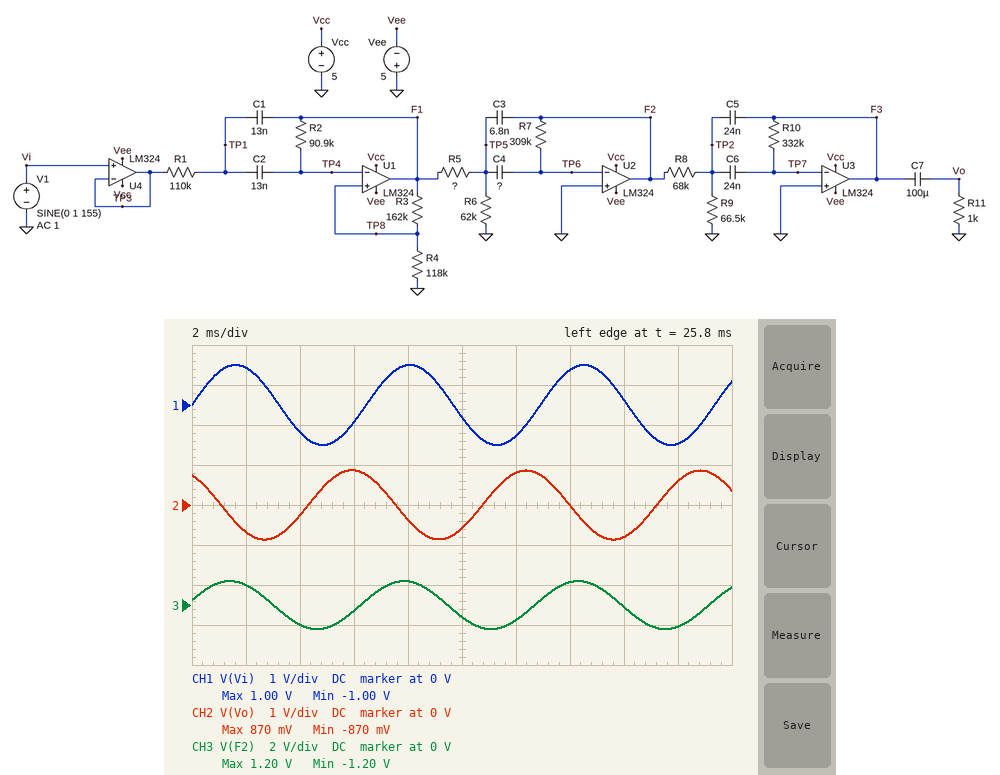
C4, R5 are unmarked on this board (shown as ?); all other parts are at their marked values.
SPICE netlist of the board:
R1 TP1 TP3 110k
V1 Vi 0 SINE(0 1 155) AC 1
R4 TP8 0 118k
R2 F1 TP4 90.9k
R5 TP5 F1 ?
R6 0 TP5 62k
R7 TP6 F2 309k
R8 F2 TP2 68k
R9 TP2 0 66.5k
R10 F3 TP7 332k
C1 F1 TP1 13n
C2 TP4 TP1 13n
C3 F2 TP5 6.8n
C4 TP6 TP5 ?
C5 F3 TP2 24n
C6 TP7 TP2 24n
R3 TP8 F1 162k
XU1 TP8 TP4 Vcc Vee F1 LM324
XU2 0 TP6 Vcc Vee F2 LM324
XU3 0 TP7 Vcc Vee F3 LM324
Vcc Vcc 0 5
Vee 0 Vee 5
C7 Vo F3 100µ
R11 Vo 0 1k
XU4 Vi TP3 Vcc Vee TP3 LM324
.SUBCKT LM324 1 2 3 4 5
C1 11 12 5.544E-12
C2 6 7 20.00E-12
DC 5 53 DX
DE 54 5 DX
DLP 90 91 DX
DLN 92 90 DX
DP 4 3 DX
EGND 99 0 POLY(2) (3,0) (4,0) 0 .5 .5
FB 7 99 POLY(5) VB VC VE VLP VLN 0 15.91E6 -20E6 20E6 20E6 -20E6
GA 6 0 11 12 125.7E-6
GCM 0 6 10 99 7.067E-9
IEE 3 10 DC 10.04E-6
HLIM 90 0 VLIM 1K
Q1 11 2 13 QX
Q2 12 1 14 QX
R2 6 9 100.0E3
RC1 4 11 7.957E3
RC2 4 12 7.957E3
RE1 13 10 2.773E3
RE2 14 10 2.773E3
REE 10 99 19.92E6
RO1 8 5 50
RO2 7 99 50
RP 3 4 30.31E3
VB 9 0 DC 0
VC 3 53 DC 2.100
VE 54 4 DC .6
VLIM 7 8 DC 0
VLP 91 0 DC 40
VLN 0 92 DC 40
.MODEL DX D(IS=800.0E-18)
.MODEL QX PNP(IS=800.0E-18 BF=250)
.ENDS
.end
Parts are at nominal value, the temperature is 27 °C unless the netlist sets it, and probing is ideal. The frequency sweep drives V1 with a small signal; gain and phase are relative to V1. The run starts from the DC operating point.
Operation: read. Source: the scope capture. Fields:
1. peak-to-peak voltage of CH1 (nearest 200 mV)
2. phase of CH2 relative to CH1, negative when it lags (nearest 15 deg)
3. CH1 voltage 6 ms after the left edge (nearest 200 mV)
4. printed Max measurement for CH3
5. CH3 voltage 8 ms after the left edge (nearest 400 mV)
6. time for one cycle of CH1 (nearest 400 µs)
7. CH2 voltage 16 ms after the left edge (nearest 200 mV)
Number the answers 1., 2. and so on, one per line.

1. 2.0 V
2. 120 deg
3. -400 mV
4. 1.20 V
5. 1.2 V
6. 6.4 ms
7. -800 mV
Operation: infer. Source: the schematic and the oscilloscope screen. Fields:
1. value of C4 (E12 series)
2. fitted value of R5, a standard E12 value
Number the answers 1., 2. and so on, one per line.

1. 8.2 nF
2. 120 kΩ
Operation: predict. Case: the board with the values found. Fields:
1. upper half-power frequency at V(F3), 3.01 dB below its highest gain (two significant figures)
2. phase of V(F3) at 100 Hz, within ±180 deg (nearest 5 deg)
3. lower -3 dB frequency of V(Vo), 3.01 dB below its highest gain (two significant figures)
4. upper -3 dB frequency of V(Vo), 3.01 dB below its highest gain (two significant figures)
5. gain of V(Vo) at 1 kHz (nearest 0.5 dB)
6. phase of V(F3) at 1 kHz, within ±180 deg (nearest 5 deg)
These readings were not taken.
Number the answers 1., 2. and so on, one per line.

1. 200 Hz
2. -160 deg
3. 61 Hz
4. 200 Hz
5. -48.5 dB
6. -70 deg
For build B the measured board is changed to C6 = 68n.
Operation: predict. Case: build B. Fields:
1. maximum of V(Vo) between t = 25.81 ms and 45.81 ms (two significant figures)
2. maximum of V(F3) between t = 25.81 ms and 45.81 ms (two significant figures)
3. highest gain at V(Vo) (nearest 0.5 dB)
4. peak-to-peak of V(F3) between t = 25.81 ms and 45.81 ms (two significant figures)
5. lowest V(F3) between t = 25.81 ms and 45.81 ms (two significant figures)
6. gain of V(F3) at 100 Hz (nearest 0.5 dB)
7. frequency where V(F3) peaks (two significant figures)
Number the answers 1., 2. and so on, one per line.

1. 790 mV
2. 780 mV
3. -2.0 dB
4. 1.6 V
5. -800 mV
6. -3.0 dB
7. 140 Hz
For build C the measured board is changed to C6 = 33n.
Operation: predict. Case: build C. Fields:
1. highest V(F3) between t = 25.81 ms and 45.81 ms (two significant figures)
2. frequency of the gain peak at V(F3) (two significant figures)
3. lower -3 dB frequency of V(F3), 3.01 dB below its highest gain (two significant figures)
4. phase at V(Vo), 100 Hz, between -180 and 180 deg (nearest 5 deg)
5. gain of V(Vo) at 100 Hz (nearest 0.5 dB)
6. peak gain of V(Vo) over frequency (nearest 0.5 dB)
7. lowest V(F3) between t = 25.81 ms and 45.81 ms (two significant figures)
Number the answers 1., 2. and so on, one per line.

1. 830 mV
2. 140 Hz
3. 55 Hz
4. -165 deg
5. -2.0 dB
6. -1.5 dB
7. -850 mV
